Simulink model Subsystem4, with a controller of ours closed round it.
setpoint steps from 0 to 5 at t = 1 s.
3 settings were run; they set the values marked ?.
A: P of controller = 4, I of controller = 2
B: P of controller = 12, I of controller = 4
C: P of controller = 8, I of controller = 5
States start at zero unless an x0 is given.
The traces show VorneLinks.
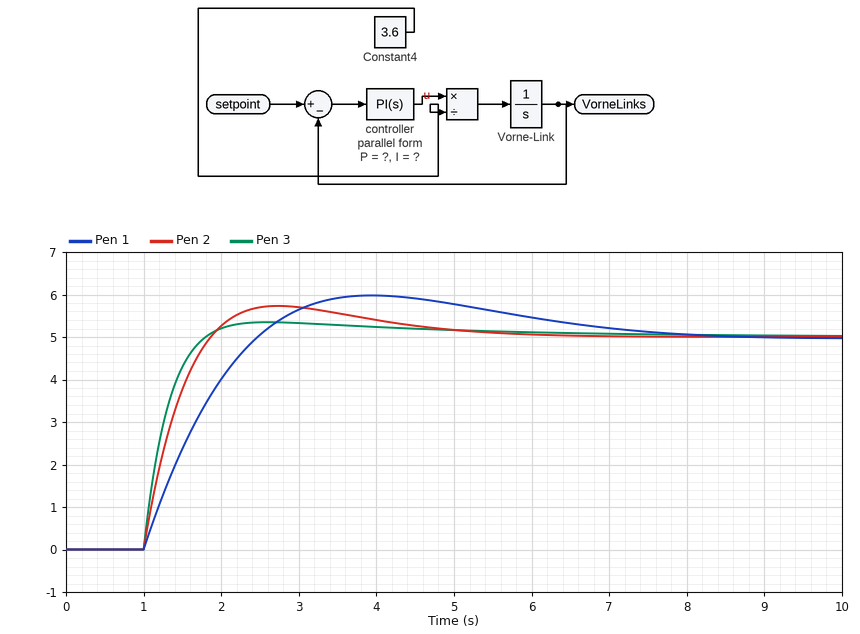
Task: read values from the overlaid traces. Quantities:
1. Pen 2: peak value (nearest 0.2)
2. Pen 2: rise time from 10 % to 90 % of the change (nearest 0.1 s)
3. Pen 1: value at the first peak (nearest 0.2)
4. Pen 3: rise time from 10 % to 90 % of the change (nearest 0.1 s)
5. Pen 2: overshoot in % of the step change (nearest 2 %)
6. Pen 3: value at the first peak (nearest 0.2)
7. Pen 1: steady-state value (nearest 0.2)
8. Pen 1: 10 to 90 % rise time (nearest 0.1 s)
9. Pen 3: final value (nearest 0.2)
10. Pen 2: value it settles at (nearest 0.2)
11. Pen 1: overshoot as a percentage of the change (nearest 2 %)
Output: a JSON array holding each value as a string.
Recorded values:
["5.8", "0.6 s", "6.0", "0.5 s", "14 %", "5.4", "5.0", "1.1 s", "5.0", "5.0", "20 %"]
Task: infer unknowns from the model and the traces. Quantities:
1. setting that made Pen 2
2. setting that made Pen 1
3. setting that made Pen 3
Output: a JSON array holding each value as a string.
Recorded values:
["C", "A", "B"]
